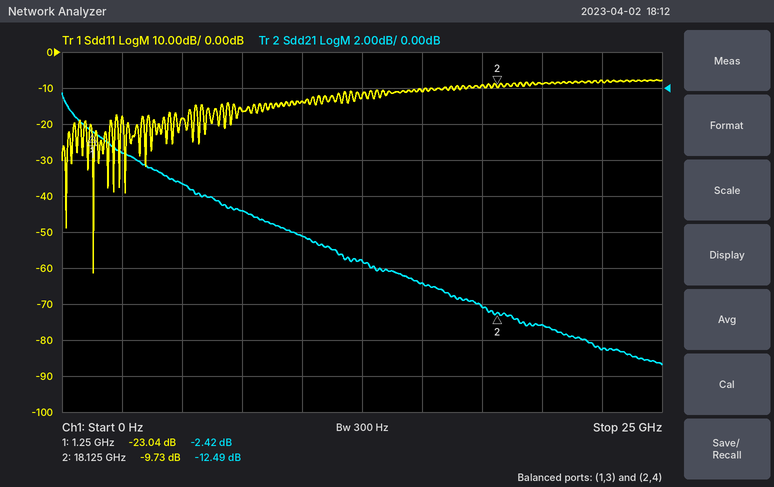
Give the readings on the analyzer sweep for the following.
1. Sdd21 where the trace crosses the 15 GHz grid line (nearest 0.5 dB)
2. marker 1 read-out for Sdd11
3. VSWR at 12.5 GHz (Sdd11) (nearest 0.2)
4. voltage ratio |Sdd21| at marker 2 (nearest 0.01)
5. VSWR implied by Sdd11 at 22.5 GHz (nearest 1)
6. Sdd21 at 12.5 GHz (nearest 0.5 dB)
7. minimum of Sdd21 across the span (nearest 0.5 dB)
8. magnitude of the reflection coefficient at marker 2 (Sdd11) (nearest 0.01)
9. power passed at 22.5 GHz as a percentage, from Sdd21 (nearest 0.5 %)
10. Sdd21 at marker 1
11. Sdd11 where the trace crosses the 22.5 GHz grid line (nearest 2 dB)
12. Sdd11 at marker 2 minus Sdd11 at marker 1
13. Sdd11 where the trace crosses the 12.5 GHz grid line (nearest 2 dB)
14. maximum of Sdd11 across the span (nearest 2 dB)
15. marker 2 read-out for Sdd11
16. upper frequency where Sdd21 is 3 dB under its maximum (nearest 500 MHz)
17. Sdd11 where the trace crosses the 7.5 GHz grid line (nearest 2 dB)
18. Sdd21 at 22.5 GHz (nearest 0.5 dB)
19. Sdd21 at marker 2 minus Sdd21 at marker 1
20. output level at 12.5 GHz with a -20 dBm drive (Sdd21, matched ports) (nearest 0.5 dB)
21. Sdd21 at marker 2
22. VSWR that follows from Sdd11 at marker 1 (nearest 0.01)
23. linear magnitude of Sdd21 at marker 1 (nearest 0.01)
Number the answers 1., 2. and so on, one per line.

1. -11.0 dB
2. -23.04 dB
3. 1.6
4. 0.24
5. 2
6. -9.5 dB
7. -15.5 dB
8. 0.33
9. 3.5 %
10. -2.42 dB
11. -8 dB
12. 13.31 dB
13. -12 dB
14. -8 dB
15. -9.73 dB
16. 2.0 GHz
17. -16 dB
18. -14.5 dB
19. -10.07 dB
20. -29.5 dBm
21. -12.49 dB
22. 1.15
23. 0.76
